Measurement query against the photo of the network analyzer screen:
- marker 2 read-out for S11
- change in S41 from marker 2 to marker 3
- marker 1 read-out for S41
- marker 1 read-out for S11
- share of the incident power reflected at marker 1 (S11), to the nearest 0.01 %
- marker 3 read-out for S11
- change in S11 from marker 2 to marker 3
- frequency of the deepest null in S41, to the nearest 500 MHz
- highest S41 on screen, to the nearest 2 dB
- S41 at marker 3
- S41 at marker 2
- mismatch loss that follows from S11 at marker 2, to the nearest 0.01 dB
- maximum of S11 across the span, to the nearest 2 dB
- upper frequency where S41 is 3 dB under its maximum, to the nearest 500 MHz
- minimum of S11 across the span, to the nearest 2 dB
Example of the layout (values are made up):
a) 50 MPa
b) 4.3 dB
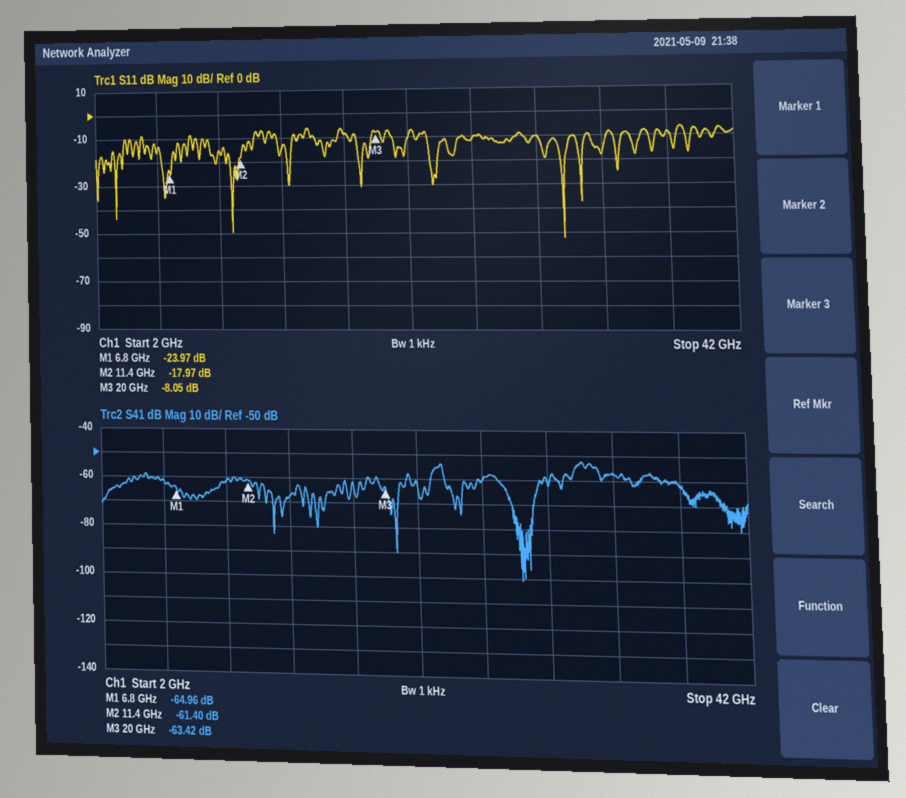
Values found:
a) -17.97 dB
b) -2.02 dB
c) -64.96 dB
d) -23.97 dB
e) 0.40 %
f) -8.05 dB
g) 9.92 dB
h) 28.5 GHz
i) -52 dB
j) -63.42 dB
k) -61.40 dB
l) 0.07 dB
m) -6 dB
n) 33.0 GHz
o) -52 dB
